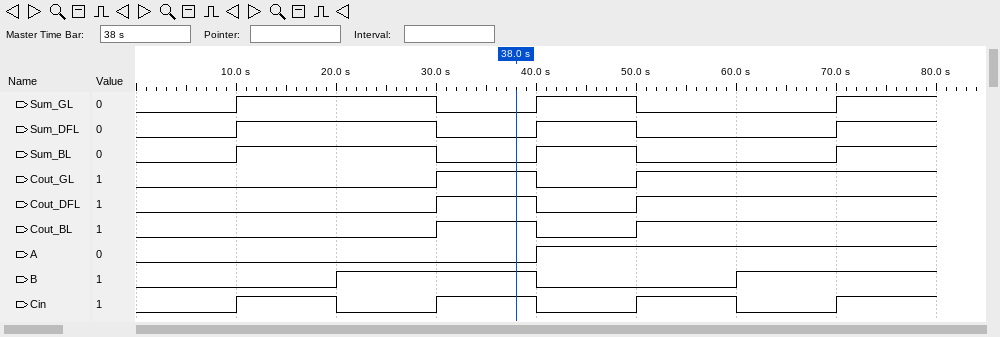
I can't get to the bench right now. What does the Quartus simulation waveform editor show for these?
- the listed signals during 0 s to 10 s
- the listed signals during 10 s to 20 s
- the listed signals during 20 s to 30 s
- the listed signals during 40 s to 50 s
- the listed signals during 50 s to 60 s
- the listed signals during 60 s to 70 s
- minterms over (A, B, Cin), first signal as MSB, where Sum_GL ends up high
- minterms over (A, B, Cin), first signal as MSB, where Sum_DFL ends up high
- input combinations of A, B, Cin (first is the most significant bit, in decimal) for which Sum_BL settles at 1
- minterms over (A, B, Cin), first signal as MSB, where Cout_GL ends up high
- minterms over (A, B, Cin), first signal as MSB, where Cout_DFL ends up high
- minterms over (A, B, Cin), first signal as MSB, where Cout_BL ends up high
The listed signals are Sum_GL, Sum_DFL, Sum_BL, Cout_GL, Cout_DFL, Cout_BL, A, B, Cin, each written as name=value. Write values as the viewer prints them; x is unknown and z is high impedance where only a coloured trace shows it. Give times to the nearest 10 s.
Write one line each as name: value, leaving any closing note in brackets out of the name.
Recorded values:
the listed signals during 0 s to 10 s: Sum_GL=0, Sum_DFL=0, Sum_BL=0, Cout_GL=0, Cout_DFL=0, Cout_BL=0, A=0, B=0, Cin=0
the listed signals during 10 s to 20 s: Sum_GL=1, Sum_DFL=1, Sum_BL=1, Cout_GL=0, Cout_DFL=0, Cout_BL=0, A=0, B=0, Cin=1
the listed signals during 20 s to 30 s: Sum_GL=1, Sum_DFL=1, Sum_BL=1, Cout_GL=0, Cout_DFL=0, Cout_BL=0, A=0, B=1, Cin=0
the listed signals during 40 s to 50 s: Sum_GL=1, Sum_DFL=1, Sum_BL=1, Cout_GL=0, Cout_DFL=0, Cout_BL=0, A=1, B=0, Cin=0
the listed signals during 50 s to 60 s: Sum_GL=0, Sum_DFL=0, Sum_BL=0, Cout_GL=1, Cout_DFL=1, Cout_BL=1, A=1, B=0, Cin=1
the listed signals during 60 s to 70 s: Sum_GL=0, Sum_DFL=0, Sum_BL=0, Cout_GL=1, Cout_DFL=1, Cout_BL=1, A=1, B=1, Cin=0
minterms over (A, B, Cin), first signal as MSB, where Sum_GL ends up high: 1, 2, 4, 7
minterms over (A, B, Cin), first signal as MSB, where Sum_DFL ends up high: 1, 2, 4, 7
input combinations of A, B, Cin (first is the most significant bit, in decimal) for which Sum_BL settles at 1: 1, 2, 4, 7
minterms over (A, B, Cin), first signal as MSB, where Cout_GL ends up high: 3, 5, 6, 7
minterms over (A, B, Cin), first signal as MSB, where Cout_DFL ends up high: 3, 5, 6, 7
minterms over (A, B, Cin), first signal as MSB, where Cout_BL ends up high: 3, 5, 6, 7
